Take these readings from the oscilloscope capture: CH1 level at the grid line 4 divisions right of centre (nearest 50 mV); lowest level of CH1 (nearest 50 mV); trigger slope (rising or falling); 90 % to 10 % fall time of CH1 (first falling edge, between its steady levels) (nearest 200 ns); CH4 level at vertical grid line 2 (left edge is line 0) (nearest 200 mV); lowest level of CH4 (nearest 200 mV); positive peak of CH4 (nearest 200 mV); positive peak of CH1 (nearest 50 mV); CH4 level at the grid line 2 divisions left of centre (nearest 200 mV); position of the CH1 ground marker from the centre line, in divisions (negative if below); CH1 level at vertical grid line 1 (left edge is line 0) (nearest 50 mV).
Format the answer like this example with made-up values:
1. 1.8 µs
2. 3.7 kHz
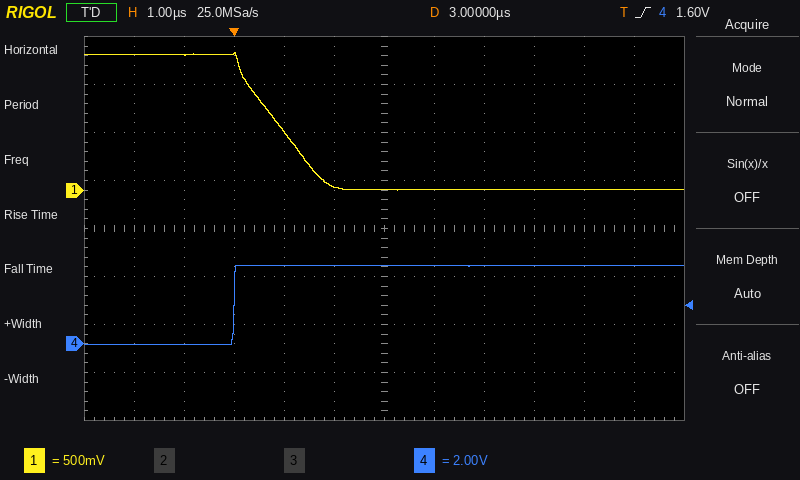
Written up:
1. 0 mV
2. 0 mV
3. rising
4. 1.6 µs
5. 0.0 V
6. 0.0 V
7. 3.2 V
8. 1.45 V
9. 3.2 V
10. +0.8 div
11. 1.40 V
